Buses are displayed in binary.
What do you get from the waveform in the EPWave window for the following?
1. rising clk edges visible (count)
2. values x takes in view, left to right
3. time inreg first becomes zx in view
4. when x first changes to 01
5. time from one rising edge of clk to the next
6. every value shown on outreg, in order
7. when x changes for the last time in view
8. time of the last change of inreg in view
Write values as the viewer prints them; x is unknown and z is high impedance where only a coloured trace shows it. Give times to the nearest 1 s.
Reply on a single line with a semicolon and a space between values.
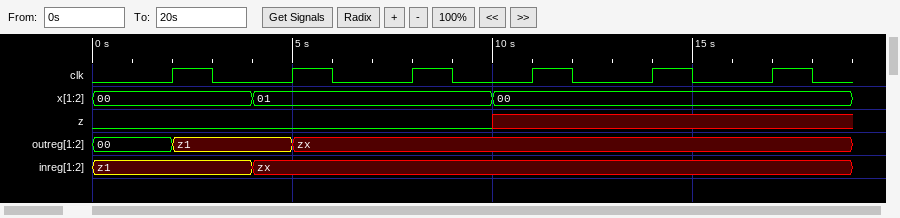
6; 00, 01, 00; 4 s; 4 s; 3 s; 00, z1, zx; 10 s; 4 s
